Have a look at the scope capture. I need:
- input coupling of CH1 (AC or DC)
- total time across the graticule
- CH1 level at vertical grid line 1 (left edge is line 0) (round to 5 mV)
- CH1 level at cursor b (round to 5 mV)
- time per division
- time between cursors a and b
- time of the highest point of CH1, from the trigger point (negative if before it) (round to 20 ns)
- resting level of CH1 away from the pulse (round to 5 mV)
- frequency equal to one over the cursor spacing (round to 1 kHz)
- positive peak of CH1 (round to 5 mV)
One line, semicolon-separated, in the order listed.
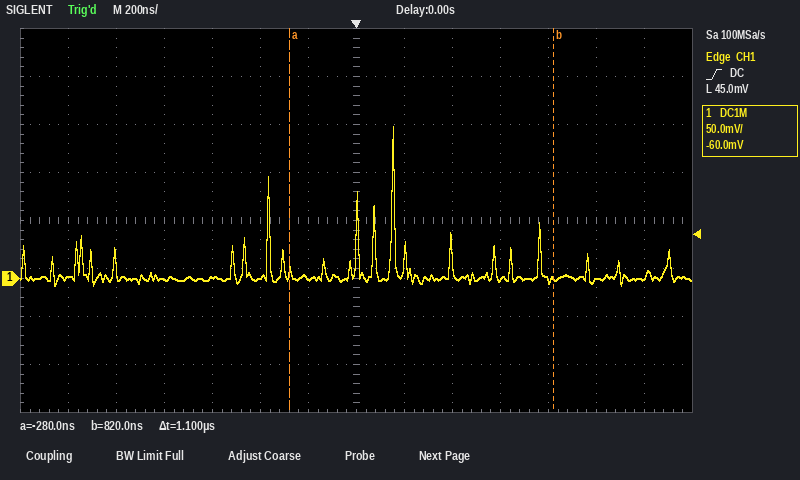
DC; 2.8 µs; 0 mV; 0 mV; 200 ns; 1.1 µs; +160 ns; 0 mV; 909 kHz; 160 mV
